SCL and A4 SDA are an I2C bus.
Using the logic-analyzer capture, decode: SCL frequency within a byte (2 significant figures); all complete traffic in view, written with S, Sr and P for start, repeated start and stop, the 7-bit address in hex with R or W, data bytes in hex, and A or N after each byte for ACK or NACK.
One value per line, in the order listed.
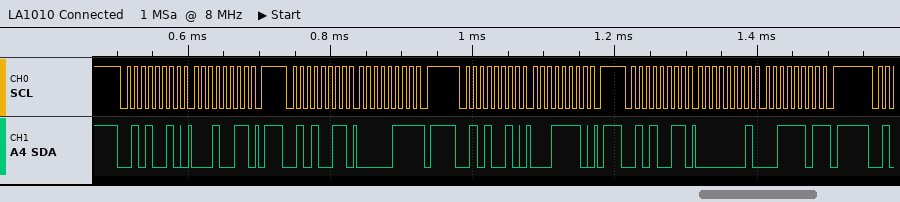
100 kHz
S 29W A 13 A P S 29R A 07 N P S 29W A 1E A P S 29R A 01 A 3D N P
